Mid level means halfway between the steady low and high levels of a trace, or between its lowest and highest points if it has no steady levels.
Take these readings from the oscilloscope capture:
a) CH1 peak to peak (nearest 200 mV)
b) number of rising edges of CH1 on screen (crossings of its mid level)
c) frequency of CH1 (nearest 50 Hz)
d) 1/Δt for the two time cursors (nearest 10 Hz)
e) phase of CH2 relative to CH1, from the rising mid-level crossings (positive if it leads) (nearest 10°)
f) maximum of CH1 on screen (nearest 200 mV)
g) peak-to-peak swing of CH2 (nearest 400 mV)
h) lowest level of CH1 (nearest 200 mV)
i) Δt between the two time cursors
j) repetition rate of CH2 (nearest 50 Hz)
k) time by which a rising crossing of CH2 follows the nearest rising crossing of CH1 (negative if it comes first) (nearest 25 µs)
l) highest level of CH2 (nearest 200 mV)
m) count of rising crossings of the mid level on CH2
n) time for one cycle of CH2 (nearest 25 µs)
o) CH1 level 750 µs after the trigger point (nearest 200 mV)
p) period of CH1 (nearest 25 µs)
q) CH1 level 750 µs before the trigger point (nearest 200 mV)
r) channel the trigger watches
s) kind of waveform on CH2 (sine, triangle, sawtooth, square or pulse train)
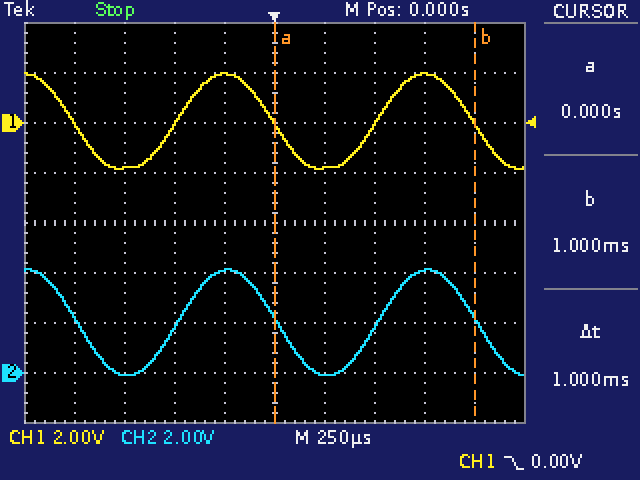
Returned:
3.8 V
2
1.00 kHz
1.00 kHz
0°
2.0 V
4.4 V
-1.8 V
1 ms
1.00 kHz
0 µs
4.2 V
2
1.000 ms
2.0 V
1.000 ms
-1.8 V
CH1
sine
